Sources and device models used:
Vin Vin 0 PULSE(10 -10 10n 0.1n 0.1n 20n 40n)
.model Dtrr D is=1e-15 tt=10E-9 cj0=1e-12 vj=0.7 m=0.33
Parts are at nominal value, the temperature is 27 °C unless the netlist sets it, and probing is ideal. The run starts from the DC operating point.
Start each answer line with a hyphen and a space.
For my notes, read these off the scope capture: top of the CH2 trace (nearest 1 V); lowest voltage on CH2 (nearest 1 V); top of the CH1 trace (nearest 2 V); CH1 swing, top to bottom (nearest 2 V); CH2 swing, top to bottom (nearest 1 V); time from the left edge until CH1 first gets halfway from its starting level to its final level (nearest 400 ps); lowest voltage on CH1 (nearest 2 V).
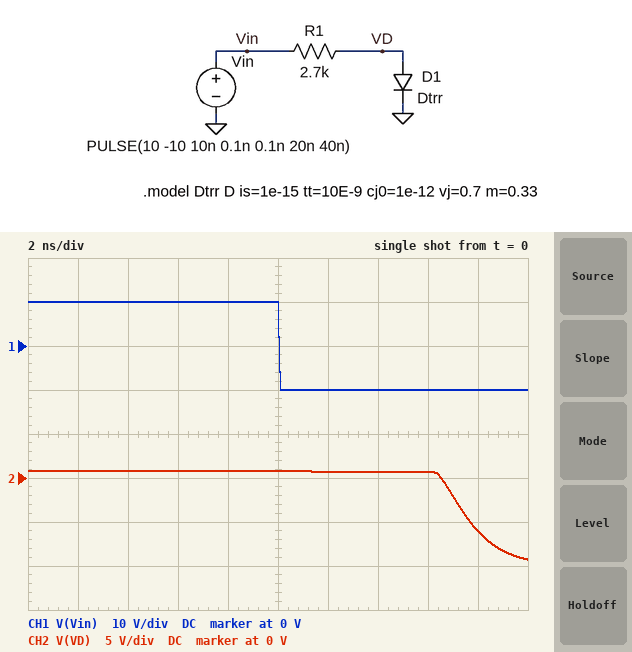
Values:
- 1 V
- -9 V
- 10 V
- 20 V
- 10 V
- 10.0 ns
- -10 V
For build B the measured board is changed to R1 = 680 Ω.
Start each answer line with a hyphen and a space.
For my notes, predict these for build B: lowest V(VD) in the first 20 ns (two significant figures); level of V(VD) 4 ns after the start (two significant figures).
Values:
- -10 V
- 780 mV
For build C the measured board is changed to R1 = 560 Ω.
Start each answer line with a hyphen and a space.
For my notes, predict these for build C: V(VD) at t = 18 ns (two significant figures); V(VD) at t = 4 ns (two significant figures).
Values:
- -10 V
- 790 mV
